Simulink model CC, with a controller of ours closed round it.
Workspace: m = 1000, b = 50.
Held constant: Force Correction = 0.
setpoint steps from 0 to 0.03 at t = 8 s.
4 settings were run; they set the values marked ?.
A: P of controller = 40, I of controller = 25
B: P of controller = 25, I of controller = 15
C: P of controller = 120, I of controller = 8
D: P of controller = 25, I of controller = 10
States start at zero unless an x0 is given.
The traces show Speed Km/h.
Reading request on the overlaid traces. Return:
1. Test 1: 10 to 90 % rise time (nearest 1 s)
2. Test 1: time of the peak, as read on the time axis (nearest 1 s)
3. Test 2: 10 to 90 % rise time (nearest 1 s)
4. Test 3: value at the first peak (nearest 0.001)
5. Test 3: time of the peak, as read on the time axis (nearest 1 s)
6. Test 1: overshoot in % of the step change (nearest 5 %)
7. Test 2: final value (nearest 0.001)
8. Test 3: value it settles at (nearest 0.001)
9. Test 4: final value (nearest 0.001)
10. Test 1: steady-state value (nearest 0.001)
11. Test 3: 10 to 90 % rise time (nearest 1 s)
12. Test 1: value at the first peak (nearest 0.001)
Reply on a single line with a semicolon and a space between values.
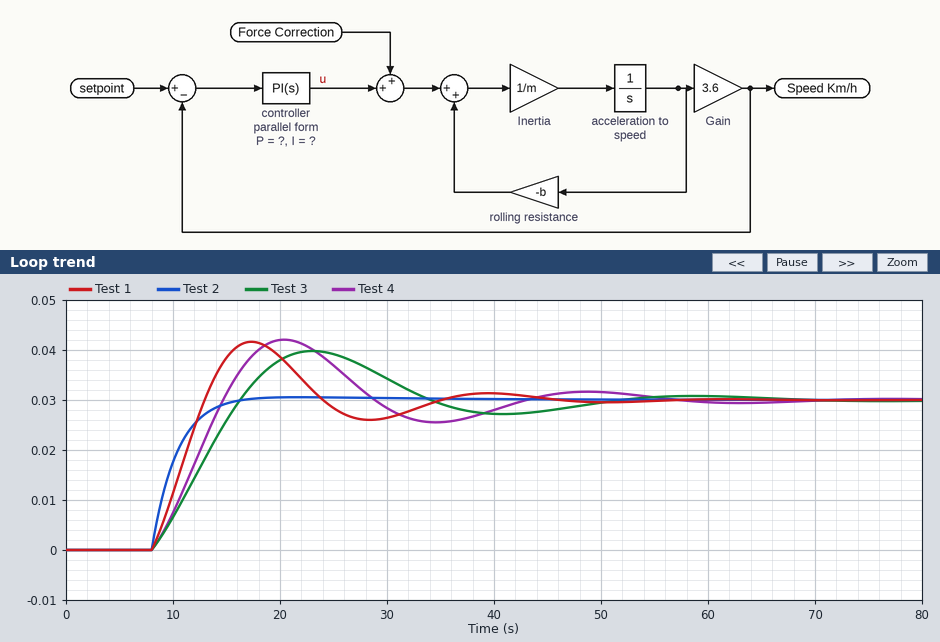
4 s; 17 s; 5 s; 0.040; 23 s; 40 %; 0.030; 0.030; 0.030; 0.030; 6 s; 0.042
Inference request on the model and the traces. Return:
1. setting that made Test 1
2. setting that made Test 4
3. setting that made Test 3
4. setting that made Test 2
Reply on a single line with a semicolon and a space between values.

A; B; D; C
